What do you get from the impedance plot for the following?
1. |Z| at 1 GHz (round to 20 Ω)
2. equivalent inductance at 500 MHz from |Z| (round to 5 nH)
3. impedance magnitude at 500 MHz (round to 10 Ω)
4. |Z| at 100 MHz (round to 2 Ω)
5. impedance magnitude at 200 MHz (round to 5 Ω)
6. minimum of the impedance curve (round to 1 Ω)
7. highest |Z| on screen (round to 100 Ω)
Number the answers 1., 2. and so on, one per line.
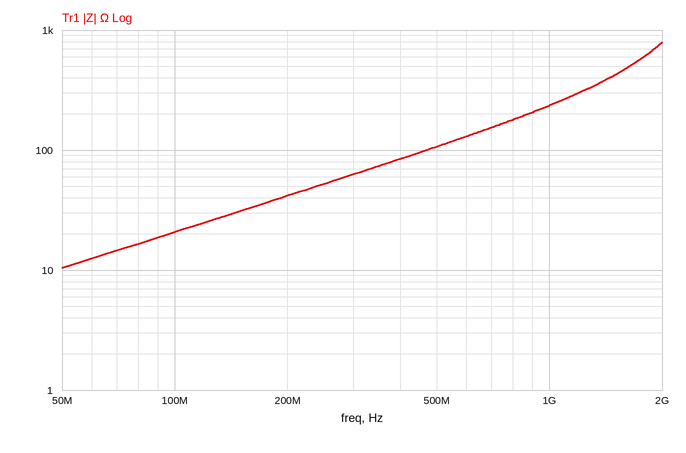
1. 240 Ω
2. 35 nH
3. 110 Ω
4. 20 Ω
5. 40 Ω
6. 10 Ω
7. 800 Ω
